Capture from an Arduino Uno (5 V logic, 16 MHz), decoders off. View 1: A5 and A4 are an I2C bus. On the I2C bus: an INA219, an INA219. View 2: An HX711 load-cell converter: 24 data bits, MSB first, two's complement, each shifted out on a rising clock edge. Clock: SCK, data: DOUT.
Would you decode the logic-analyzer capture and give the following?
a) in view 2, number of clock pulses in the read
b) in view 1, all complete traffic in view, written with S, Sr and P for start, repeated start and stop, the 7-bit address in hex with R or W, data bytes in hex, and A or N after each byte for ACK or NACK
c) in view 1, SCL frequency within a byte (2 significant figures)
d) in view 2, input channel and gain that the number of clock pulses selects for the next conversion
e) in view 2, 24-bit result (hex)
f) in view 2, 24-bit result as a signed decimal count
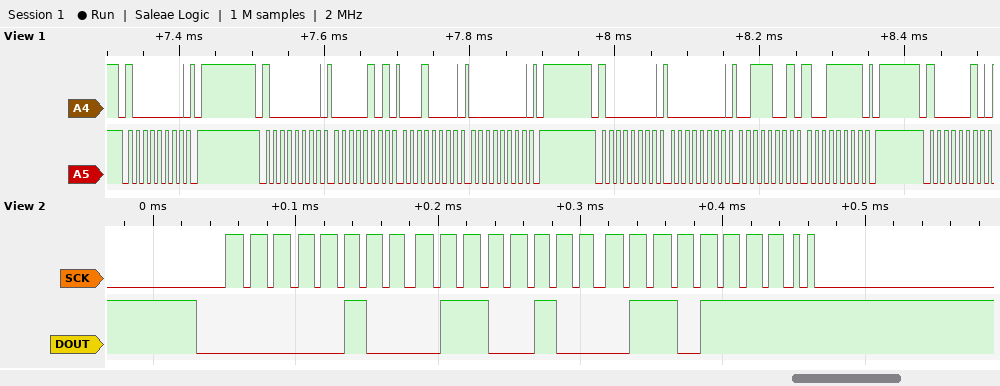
26
S 40W A P S 40W A 05 A 10 A 00 A P S 40W A 00 A 39 A 9F A P S 41W A
100 kHz
channel B, gain 32
0x04646F
287855
